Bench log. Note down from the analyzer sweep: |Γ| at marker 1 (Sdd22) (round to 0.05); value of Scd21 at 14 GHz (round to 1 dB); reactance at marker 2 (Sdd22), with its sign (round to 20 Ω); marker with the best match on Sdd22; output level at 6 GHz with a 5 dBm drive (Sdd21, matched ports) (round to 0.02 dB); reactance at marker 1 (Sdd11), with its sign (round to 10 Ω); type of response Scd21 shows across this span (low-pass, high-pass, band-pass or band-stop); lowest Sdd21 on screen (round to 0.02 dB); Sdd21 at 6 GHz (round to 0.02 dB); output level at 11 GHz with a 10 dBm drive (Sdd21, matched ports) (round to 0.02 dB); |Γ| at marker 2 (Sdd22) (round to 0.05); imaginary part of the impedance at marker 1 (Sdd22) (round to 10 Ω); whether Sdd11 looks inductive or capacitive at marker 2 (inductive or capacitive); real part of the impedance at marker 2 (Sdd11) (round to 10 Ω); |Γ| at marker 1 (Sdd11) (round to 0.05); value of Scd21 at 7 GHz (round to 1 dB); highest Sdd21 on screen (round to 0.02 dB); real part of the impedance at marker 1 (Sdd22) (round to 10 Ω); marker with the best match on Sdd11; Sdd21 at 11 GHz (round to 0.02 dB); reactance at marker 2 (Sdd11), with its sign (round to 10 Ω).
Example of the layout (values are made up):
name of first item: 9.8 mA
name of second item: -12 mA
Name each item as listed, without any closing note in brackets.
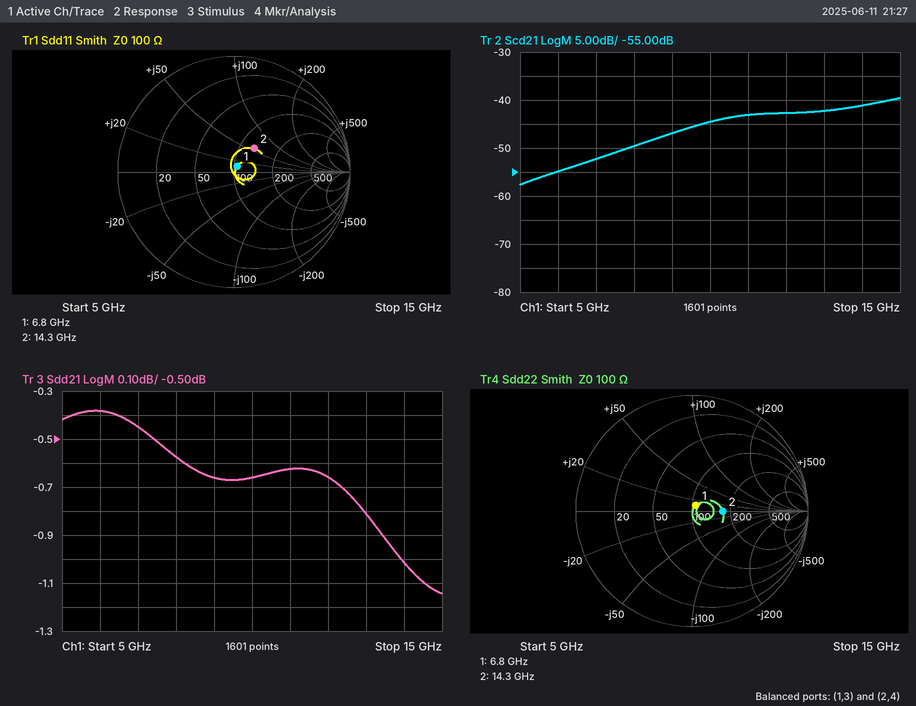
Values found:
|Γ| at marker 1 (Sdd22): 0.05
value of Scd21 at 14 GHz: -41 dB
reactance at marker 2 (Sdd22), with its sign: 0 Ω
marker with the best match on Sdd22: marker 1
output level at 6 GHz with a 5 dBm drive (Sdd21, matched ports): 4.62 dBm
reactance at marker 1 (Sdd11), with its sign: +10 Ω
type of response Scd21 shows across this span: high-pass
lowest Sdd21 on screen: -1.14 dB
Sdd21 at 6 GHz: -0.38 dB
output level at 11 GHz with a 10 dBm drive (Sdd21, matched ports): 9.38 dBm
|Γ| at marker 2 (Sdd22): 0.25
imaginary part of the impedance at marker 1 (Sdd22): +10 Ω
whether Sdd11 looks inductive or capacitive at marker 2: inductive
real part of the impedance at marker 2 (Sdd11): 130 Ω
|Γ| at marker 1 (Sdd11): 0.05
value of Scd21 at 7 GHz: -52 dB
highest Sdd21 on screen: -0.38 dB
real part of the impedance at marker 1 (Sdd22): 110 Ω
marker with the best match on Sdd11: marker 1
Sdd21 at 11 GHz: -0.62 dB
reactance at marker 2 (Sdd11), with its sign: +60 Ω
